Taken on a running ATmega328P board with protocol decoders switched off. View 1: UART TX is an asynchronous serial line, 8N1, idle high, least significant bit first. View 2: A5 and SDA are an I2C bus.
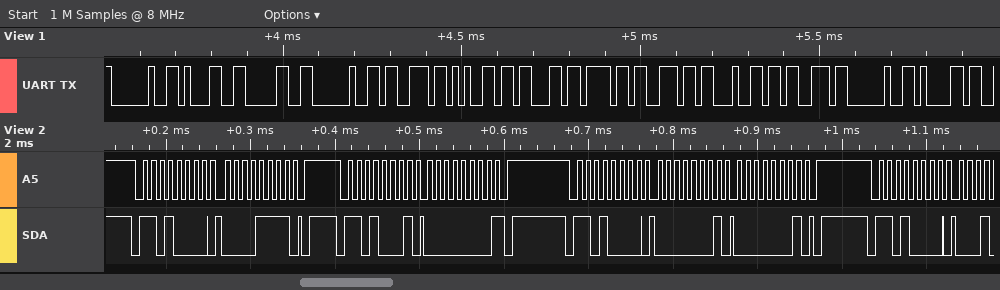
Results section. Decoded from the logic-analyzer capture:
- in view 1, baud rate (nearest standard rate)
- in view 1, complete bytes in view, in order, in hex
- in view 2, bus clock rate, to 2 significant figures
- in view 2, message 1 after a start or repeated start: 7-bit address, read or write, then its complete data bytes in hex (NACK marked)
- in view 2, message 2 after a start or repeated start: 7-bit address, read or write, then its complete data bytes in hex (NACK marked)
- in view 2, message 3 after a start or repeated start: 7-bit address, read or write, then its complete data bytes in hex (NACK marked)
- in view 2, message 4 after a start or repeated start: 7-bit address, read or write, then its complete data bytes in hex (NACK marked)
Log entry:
57600 baud
0x20 0x31 0x30 0x20 0x73 0x65 0x63 0x6F 0x6E 0x64 0x73 0x20 0x61
100 kHz
0x68 write: 0F
0x68 read: 00 NACK
0x68 write: 01 01
0x68 write
